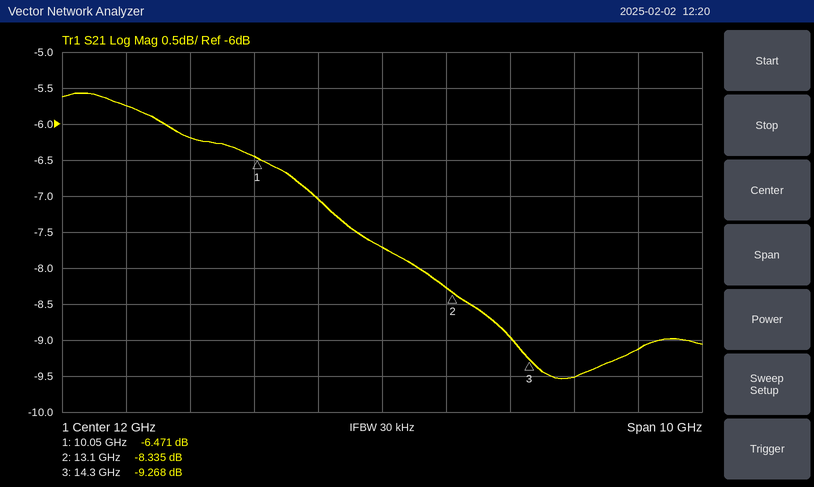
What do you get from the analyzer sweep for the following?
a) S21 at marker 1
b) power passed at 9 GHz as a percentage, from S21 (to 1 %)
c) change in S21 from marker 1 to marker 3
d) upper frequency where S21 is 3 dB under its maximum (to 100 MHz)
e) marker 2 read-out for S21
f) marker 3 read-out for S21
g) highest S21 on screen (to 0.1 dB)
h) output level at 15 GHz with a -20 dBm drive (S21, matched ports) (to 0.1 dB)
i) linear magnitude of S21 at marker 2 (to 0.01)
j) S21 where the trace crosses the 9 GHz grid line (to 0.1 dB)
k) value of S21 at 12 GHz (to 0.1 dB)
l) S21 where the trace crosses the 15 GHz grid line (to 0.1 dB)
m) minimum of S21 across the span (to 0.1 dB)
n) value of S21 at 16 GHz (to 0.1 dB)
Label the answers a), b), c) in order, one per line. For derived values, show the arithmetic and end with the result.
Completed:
a) -6.471 dB
b) 10^(-6.2/10) ≈ 24 %
c) -9.268 − (-6.471) = -2.797 dB
d) 13.5 GHz
e) -8.335 dB
f) -9.268 dB
g) -5.6 dB
h) -20 dBm + (-9.5 dB) = -29.5 dBm
i) 10^(-8.335/20) ≈ 0.38
j) -6.2 dB
k) -7.7 dB
l) -9.5 dB
m) -9.5 dB
n) -9.1 dB
